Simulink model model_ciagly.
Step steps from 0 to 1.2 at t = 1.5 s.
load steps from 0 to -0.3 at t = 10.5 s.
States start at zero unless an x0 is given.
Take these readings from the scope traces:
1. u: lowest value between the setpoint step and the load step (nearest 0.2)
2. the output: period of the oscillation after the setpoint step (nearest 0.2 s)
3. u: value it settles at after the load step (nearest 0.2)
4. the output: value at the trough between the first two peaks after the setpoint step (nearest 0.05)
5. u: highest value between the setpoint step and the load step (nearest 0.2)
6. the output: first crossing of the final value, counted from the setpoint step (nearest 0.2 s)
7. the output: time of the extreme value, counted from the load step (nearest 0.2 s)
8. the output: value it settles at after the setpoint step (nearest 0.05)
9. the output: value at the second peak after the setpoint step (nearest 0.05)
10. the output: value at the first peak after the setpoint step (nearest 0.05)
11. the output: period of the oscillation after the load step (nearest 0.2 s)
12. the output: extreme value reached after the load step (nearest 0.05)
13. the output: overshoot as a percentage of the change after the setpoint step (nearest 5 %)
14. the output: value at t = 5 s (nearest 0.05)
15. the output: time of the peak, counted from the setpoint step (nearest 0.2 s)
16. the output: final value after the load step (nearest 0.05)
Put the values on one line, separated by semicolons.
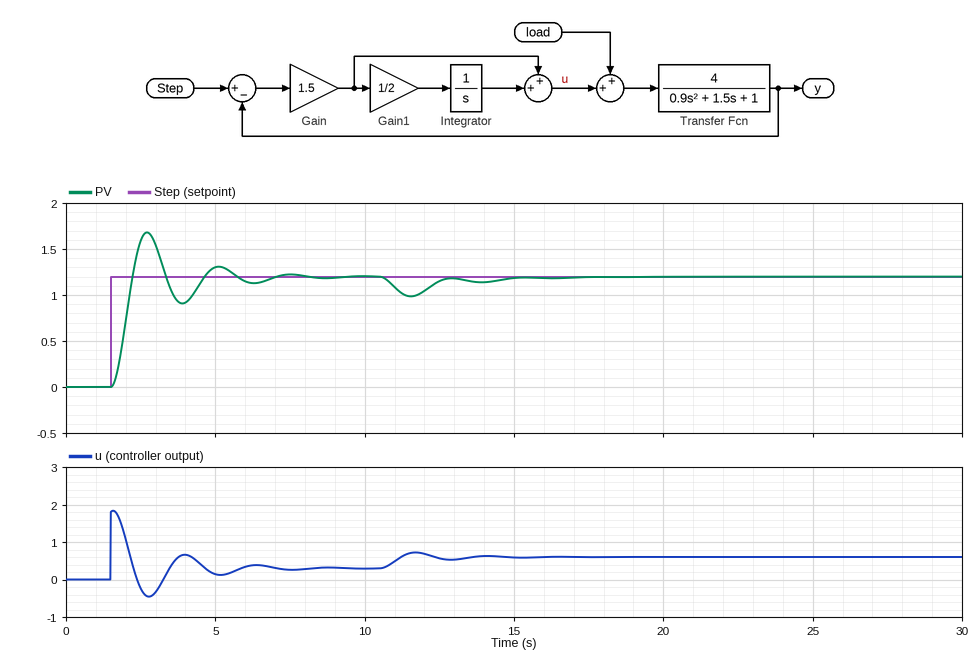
-0.4; 2.4 s; 0.6; 0.90; 1.8; 0.8 s; 1.0 s; 1.20; 1.30; 1.70; 2.4 s; 1.00; 40 %; 1.30; 1.2 s; 1.20
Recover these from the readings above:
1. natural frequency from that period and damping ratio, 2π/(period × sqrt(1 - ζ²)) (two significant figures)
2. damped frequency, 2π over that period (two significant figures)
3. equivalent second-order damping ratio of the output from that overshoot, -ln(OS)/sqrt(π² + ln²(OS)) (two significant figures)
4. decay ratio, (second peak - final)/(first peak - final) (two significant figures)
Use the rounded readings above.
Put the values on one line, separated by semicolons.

2.7 rad/s; 2.6 rad/s; 0.28; 0.20
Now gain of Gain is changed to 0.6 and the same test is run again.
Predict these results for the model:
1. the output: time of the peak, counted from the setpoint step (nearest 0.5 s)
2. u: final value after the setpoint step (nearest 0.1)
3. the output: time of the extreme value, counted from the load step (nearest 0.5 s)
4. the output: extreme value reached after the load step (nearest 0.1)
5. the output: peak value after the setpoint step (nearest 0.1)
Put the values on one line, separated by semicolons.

2.0 s; 0.3; 1.5 s; 0.8; 1.4
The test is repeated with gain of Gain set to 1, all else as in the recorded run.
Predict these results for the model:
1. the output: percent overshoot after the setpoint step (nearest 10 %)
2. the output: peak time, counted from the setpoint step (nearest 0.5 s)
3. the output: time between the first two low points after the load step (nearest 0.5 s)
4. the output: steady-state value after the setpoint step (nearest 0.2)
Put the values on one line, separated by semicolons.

30 %; 1.5 s; 3.0 s; 1.2
